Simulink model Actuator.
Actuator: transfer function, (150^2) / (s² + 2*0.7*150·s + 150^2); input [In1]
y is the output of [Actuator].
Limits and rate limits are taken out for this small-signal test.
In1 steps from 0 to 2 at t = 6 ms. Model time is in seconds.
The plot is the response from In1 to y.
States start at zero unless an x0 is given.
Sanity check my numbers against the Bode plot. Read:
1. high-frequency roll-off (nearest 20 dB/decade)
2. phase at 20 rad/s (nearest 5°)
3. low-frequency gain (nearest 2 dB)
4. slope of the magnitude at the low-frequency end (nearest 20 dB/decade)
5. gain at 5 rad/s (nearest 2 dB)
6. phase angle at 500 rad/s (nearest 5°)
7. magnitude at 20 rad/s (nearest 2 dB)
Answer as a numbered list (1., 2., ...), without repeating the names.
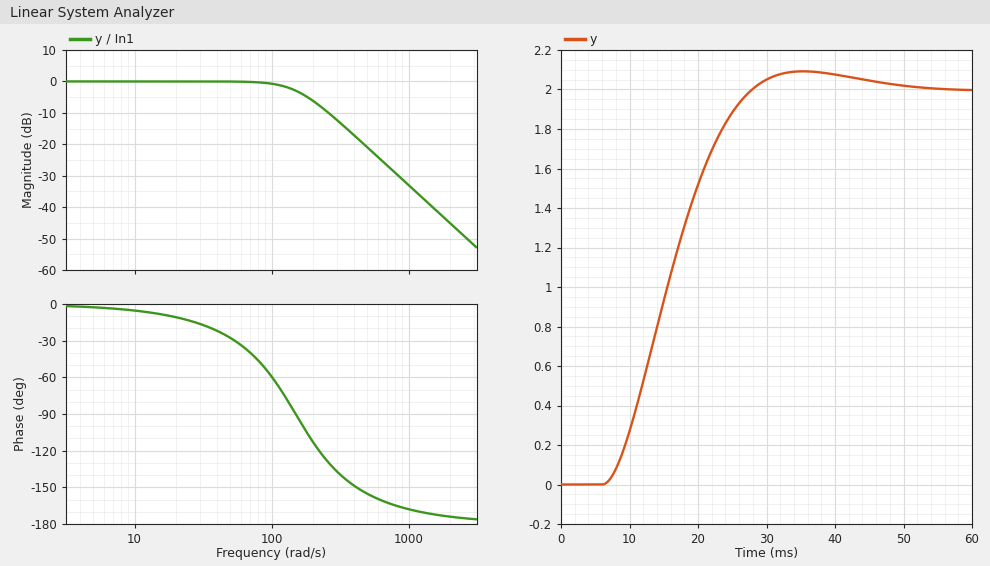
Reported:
1. -40 dB/decade
2. -10°
3. 0 dB
4. 0 dB/decade
5. 0 dB
6. -155°
7. 0 dB
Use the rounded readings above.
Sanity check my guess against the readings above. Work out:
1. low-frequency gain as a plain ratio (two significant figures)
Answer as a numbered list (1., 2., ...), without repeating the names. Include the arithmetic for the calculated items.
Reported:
1. 10^(0 / 20) = 1.0
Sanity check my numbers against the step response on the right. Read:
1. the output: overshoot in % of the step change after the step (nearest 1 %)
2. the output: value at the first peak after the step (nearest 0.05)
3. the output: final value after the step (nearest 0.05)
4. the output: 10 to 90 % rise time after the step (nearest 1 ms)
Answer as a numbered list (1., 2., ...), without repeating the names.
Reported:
1. 5 %
2. 2.10
3. 2.00
4. 14 ms
